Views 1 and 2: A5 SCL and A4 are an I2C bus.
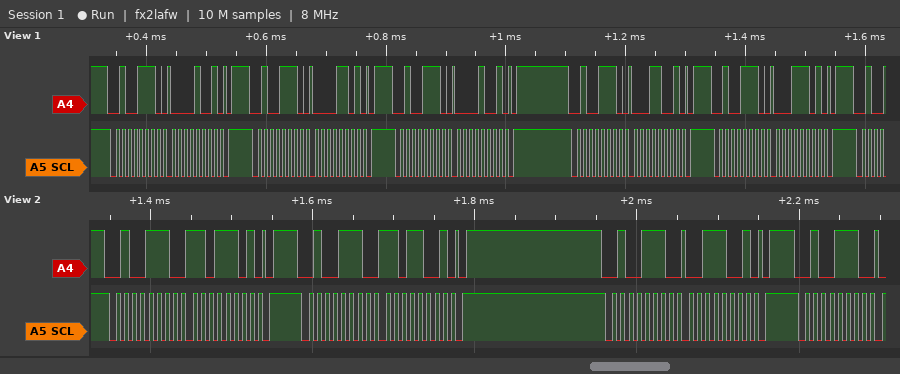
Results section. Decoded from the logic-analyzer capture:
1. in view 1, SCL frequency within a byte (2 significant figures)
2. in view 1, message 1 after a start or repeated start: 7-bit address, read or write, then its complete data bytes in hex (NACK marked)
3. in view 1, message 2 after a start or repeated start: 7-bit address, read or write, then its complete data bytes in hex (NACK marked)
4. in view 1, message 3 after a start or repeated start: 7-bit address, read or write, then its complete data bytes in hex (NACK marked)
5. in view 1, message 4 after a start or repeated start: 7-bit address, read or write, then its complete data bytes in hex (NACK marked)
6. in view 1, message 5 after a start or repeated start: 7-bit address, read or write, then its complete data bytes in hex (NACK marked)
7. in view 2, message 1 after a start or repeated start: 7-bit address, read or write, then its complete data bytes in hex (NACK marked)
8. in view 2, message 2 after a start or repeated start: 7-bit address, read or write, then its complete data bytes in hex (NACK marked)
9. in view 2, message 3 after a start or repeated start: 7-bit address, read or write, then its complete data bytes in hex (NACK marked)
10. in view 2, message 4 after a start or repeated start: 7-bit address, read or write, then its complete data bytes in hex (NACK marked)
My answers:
100 kHz
0x27 write: 09
0x27 write: 0D
0x27 write: 09
0x27 write: 19
0x27 write: 1D
0x27 write: DD
0x27 write: D9
0x27 write: 39
0x27 write
